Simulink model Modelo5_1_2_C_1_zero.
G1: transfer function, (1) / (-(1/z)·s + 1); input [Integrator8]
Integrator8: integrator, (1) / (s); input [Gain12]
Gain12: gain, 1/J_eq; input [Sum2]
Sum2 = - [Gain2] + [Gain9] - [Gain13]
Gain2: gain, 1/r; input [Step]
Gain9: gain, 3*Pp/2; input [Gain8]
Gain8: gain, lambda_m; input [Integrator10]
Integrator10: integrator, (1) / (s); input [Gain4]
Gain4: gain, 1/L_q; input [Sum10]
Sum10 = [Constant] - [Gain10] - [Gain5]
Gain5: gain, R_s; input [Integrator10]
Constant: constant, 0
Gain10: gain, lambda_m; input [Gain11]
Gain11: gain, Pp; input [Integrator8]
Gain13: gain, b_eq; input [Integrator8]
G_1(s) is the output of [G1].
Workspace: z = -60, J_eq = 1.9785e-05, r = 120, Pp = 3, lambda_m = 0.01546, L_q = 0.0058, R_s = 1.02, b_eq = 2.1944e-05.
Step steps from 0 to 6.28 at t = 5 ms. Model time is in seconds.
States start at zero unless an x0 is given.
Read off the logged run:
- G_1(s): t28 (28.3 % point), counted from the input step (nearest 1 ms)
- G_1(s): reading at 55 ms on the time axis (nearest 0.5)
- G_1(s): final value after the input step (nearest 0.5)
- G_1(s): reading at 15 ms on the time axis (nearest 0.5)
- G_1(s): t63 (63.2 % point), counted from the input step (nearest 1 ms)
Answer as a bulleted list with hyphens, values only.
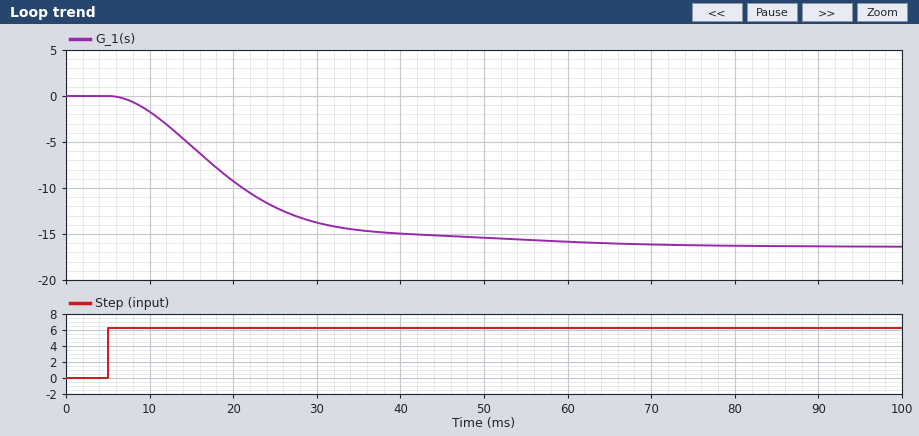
- 9 ms
- -15.5
- -16.5
- -5.5
- 17 ms
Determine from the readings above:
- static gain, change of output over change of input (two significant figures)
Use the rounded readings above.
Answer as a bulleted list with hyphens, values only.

- -2.6
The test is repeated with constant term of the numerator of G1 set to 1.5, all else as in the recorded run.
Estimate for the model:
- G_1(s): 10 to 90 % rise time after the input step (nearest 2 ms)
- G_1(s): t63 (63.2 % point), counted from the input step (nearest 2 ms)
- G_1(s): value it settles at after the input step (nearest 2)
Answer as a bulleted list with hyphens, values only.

- 28 ms
- 16 ms
- -24
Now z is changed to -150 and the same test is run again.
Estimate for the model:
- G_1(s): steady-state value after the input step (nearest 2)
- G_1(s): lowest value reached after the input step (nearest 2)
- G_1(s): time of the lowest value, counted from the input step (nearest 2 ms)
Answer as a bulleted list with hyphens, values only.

- -16
- -18
- 24 ms
